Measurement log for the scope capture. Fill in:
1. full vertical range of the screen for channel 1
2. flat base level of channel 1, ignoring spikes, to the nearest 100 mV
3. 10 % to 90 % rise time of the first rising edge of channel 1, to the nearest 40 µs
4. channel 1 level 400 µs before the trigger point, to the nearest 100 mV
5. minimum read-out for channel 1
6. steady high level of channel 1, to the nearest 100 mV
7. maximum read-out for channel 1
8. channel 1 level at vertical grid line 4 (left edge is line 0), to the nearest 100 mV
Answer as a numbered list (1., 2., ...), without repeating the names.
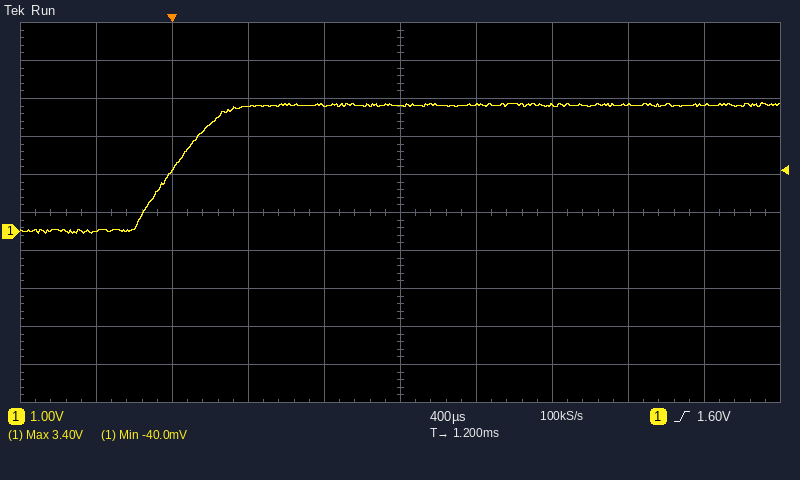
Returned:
1. 10 V
2. 0.0 V
3. 400 µs
4. 0.0 V
5. -40.0 mV
6. 3.3 V
7. 3.40 V
8. 3.3 V
